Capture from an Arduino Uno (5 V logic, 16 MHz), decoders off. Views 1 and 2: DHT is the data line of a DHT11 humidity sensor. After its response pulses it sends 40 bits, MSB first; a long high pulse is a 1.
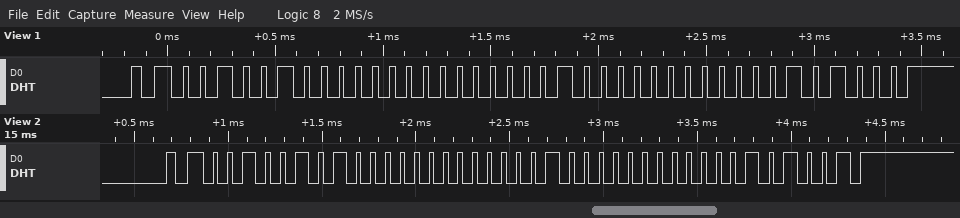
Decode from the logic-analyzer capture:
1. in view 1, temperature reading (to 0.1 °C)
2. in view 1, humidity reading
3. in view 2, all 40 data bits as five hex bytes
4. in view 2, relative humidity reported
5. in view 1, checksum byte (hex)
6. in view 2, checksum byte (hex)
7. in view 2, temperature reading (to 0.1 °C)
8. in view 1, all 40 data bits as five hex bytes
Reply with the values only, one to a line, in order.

4.0 °C
36 %
25 00 04 00 29
37 %
0x28
0x29
4.0 °C
24 00 04 00 28
